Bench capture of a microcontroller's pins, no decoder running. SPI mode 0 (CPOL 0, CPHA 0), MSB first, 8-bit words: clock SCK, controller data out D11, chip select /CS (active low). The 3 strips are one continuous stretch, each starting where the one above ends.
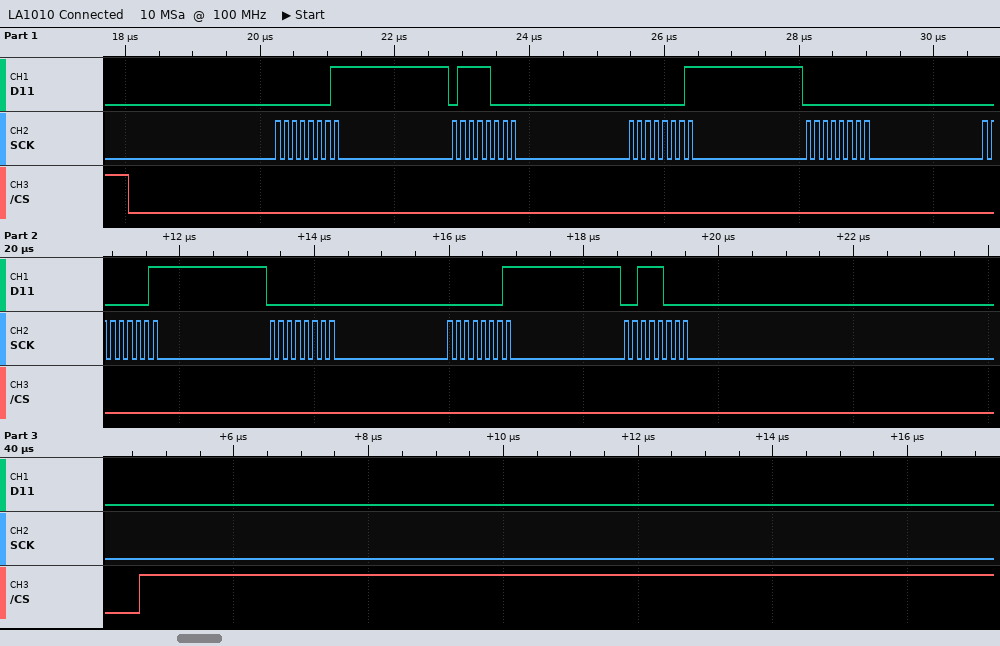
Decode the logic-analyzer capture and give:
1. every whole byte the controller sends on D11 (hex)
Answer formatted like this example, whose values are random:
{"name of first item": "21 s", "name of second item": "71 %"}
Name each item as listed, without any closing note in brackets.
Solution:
{"every whole byte the controller sends on D11": "01 78 01 00 01 00 01 38"}
